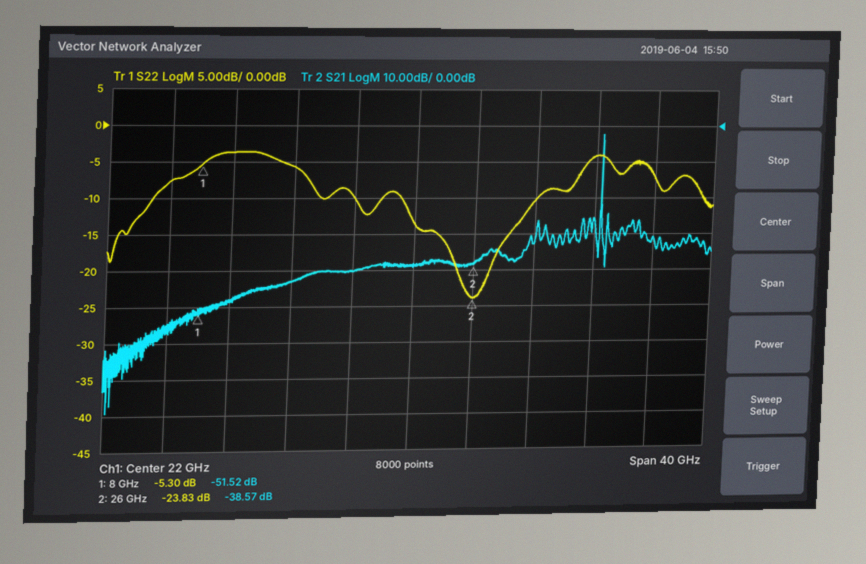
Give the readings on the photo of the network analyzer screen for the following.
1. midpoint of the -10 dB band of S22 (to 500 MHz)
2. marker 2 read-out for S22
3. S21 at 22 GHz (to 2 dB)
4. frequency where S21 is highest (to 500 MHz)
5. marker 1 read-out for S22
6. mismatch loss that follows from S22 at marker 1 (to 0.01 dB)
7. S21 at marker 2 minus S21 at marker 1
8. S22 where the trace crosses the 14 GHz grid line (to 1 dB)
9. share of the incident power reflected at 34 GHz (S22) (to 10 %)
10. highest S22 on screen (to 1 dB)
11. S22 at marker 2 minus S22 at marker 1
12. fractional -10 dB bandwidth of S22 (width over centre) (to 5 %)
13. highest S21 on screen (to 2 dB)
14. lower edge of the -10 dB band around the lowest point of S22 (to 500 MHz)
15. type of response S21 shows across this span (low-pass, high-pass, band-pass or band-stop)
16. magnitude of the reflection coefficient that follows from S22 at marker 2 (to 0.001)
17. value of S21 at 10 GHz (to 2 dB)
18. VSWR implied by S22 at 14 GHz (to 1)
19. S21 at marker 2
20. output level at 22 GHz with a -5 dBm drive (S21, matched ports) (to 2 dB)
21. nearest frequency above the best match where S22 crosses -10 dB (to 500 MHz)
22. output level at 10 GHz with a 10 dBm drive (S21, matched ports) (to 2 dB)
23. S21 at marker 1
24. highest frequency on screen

25.5 GHz
-23.83 dB
-38 dB
34.5 GHz
-5.30 dB
1.52 dB
12.95 dB
-6 dB
40 %
-4 dB
-18.53 dB
35 %
-2 dB
21.0 GHz
band-pass
0.064
-48 dB
3
-38.57 dB
-44 dBm
30.0 GHz
-38 dBm
-51.52 dB
42 GHz
